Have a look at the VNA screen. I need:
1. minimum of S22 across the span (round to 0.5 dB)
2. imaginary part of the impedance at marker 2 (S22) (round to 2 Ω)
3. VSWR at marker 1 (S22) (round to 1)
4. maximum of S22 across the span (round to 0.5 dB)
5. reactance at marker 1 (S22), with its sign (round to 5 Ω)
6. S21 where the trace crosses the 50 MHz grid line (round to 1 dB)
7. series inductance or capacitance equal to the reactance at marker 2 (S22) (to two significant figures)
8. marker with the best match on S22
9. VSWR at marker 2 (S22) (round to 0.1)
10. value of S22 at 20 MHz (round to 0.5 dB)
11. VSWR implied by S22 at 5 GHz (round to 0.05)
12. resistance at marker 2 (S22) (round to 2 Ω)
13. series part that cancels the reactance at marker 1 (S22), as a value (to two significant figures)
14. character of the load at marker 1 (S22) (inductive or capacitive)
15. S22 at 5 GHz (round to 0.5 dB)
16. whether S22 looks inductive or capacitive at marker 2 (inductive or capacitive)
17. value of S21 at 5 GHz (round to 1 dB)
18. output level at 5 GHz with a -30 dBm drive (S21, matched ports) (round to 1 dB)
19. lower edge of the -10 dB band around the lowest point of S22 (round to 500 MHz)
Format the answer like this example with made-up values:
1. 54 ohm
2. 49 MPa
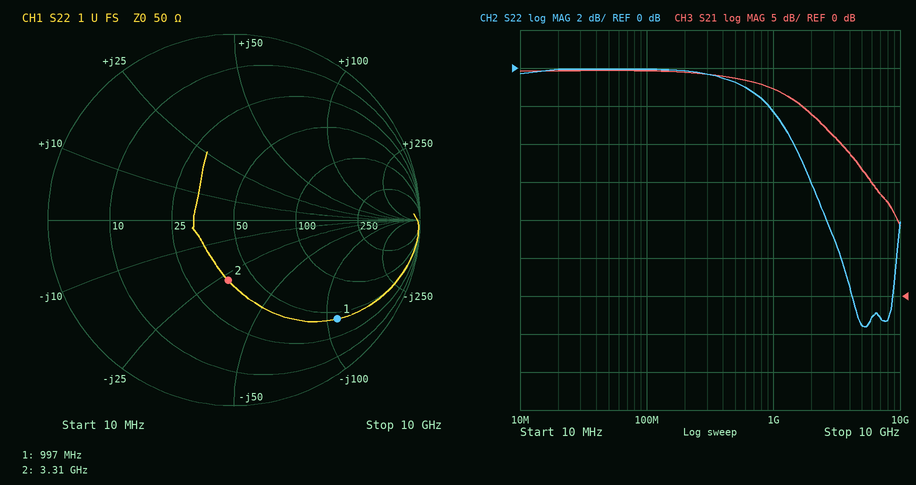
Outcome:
1. -13.5 dB
2. -28 Ω
3. 8
4. 0.0 dB
5. -110 Ω
6. 30 dB
7. 1.7 pF
8. marker 2
9. 2.0
10. 0.0 dB
11. 1.55
12. 38 Ω
13. 18 nH
14. capacitive
15. -13.5 dB
16. capacitive
17. 17 dB
18. -13 dBm
19. 3.5 GHz
